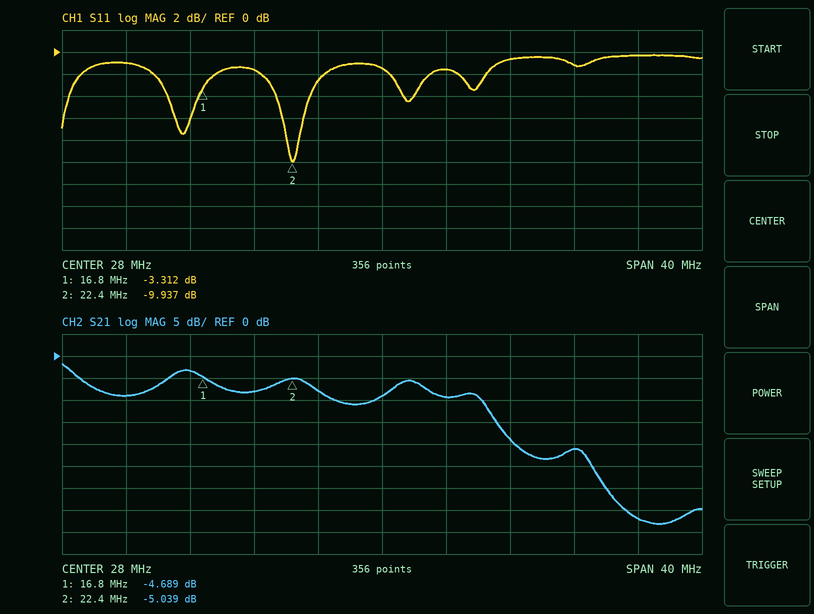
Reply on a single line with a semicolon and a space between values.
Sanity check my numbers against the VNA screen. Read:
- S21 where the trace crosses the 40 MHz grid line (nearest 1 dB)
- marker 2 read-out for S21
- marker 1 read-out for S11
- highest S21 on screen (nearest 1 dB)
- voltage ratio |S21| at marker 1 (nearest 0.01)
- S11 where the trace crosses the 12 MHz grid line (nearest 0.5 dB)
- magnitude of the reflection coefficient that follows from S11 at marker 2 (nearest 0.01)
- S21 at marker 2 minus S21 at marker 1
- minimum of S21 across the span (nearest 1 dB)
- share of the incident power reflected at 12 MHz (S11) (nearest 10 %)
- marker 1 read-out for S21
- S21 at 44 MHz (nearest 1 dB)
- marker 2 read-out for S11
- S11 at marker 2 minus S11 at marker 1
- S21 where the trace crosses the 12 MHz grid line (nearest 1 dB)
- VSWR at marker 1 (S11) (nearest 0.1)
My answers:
-21 dB; -5.039 dB; -3.312 dB; -2 dB; 0.58; -1.0 dB; 0.32; -0.350 dB; -38 dB; 80 %; -4.689 dB; -37 dB; -9.937 dB; -6.625 dB; -9 dB; 5.3
